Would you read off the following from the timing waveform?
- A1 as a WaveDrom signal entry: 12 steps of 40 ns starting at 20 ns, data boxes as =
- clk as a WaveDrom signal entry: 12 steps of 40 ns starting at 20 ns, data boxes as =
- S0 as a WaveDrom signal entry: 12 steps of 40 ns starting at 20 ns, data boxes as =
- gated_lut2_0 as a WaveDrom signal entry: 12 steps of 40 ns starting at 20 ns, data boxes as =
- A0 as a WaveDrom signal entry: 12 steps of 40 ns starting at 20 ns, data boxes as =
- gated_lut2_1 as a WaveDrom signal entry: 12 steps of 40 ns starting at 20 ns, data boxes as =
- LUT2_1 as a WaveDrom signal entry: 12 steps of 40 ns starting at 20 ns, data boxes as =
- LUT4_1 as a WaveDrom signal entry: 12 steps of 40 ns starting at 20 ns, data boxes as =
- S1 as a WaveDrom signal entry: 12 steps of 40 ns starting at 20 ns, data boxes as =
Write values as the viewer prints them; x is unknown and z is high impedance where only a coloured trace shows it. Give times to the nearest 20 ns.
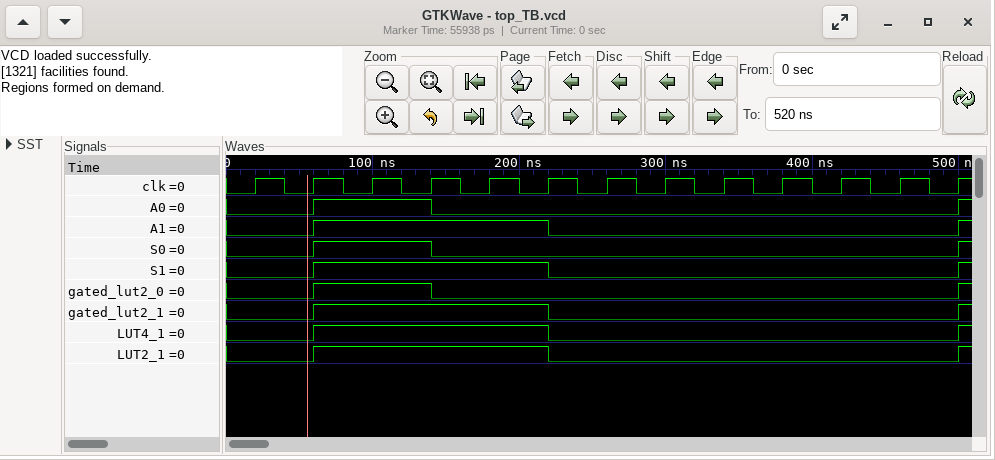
{name: 'A1', wave: '01...0......'}
{name: 'clk', wave: 'p...........'}
{name: 'S0', wave: '01.0........'}
{name: 'gated_lut2_0', wave: '01.0........'}
{name: 'A0', wave: '01.0........'}
{name: 'gated_lut2_1', wave: '01...0......'}
{name: 'LUT2_1', wave: '01...0......'}
{name: 'LUT4_1', wave: '01...0......'}
{name: 'S1', wave: '01...0......'}
